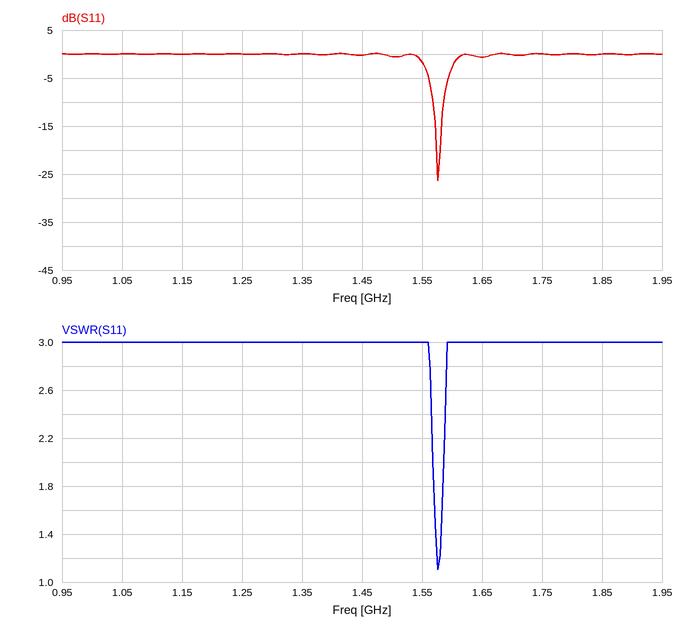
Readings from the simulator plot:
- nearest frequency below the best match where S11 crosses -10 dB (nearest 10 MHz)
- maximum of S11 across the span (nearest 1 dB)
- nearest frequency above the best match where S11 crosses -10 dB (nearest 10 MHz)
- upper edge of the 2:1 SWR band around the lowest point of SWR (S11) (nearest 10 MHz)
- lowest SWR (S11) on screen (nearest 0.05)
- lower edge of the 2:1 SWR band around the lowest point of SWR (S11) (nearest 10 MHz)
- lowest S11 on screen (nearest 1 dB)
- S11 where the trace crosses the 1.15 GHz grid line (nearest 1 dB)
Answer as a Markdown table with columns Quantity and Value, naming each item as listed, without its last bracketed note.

| Quantity | Value |
|---|---|
| nearest frequency below the best match where S11 crosses -10 dB | 1.57 GHz |
| maximum of S11 across the span | 0 dB |
| nearest frequency above the best match where S11 crosses -10 dB | 1.59 GHz |
| upper edge of the 2:1 SWR band around the lowest point of SWR (S11) | 1.59 GHz |
| lowest SWR (S11) on screen | 1.10 |
| lower edge of the 2:1 SWR band around the lowest point of SWR (S11) | 1.57 GHz |
| lowest S11 on screen | -26 dB |
| S11 where the trace crosses the 1.15 GHz grid line | 0 dB |
